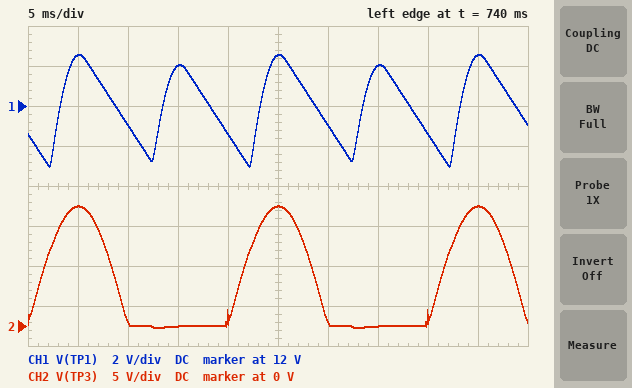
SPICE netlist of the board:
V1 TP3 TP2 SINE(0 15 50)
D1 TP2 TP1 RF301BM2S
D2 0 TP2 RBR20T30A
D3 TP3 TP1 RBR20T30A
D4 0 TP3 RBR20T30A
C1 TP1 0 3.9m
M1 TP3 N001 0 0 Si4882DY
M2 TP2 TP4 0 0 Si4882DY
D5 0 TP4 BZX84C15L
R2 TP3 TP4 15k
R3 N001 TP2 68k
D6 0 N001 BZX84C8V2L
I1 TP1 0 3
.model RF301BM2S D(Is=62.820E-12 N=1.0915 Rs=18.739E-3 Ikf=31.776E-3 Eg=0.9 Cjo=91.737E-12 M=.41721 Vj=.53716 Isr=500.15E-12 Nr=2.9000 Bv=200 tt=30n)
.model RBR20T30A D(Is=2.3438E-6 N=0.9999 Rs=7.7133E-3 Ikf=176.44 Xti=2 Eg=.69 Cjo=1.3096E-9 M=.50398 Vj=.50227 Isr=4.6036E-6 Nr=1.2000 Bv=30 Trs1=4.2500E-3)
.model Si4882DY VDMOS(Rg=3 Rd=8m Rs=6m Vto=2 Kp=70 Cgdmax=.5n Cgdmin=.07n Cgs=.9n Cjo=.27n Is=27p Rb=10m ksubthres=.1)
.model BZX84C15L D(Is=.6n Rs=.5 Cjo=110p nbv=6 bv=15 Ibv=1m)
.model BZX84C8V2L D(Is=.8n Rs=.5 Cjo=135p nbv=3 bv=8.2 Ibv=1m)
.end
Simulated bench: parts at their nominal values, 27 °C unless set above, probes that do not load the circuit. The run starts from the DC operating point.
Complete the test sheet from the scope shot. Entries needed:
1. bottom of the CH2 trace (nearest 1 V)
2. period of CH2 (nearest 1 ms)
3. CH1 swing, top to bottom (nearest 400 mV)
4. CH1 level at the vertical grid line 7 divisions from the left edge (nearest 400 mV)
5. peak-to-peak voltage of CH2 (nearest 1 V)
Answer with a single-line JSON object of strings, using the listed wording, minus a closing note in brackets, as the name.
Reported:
{"bottom of the CH2 trace": "0 V", "period of CH2": "20 ms", "CH1 swing, top to bottom": "5.6 V", "CH1 level at the vertical grid line 7 divisions from the left edge": "14.0 V", "peak-to-peak voltage of CH2": "15 V"}
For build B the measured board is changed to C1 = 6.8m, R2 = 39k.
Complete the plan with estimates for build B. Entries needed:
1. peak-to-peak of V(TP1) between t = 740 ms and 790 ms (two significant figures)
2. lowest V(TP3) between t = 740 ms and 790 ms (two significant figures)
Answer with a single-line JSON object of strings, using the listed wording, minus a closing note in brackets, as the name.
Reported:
{"peak-to-peak of V(TP1) between t = 740 ms and 790 ms": "3.7 V", "lowest V(TP3) between t = 740 ms and 790 ms": "-270 mV"}
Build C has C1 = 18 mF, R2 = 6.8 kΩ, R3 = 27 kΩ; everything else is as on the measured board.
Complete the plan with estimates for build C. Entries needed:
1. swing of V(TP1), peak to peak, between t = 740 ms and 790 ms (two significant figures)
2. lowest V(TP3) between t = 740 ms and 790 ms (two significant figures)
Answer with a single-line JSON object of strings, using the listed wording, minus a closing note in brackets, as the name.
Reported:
{"swing of V(TP1), peak to peak, between t = 740 ms and 790 ms": "1.9 V", "lowest V(TP3) between t = 740 ms and 790 ms": "-250 mV"}
